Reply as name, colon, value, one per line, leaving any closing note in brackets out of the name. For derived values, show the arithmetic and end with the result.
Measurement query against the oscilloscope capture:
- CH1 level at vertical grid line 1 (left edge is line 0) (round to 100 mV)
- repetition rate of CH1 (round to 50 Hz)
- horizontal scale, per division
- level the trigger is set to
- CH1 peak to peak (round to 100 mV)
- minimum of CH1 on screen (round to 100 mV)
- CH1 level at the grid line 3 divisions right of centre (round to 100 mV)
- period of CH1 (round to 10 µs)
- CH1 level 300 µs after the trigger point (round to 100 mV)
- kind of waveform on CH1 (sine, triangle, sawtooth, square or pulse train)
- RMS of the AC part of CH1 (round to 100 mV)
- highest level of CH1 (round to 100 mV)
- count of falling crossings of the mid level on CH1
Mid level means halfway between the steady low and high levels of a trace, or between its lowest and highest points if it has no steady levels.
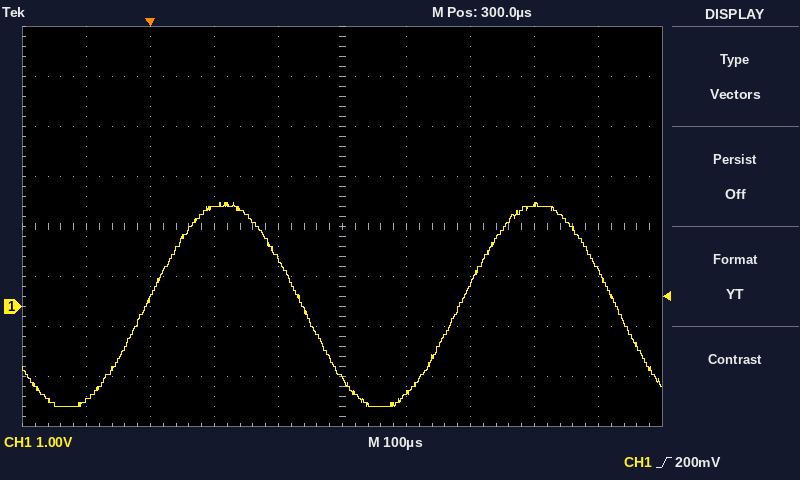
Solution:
CH1 level at vertical grid line 1 (left edge is line 0): -1.9 V
repetition rate of CH1: 1 / 490 µs ≈ 2.04 kHz, so 2.05 kHz to the nearest 50 Hz
horizontal scale, per division: 100 µs
level the trigger is set to: 200 mV
CH1 peak to peak: 2.1 V − (-2.0 V) = 4.1 V
minimum of CH1 on screen: -2.0 V
CH1 level at the grid line 3 divisions right of centre: 2.0 V
period of CH1: 490 µs
CH1 level 300 µs after the trigger point: -1.4 V
kind of waveform on CH1: sine
RMS of the AC part of CH1: 4.1 V / (2√2) ≈ 1.4 V
highest level of CH1: 2.1 V
count of falling crossings of the mid level on CH1: 2
